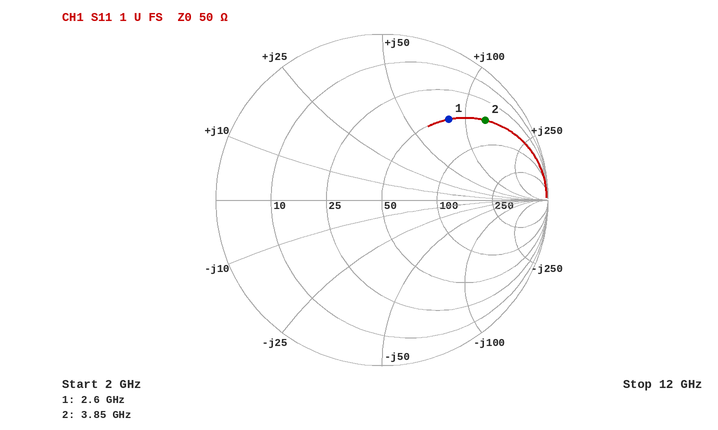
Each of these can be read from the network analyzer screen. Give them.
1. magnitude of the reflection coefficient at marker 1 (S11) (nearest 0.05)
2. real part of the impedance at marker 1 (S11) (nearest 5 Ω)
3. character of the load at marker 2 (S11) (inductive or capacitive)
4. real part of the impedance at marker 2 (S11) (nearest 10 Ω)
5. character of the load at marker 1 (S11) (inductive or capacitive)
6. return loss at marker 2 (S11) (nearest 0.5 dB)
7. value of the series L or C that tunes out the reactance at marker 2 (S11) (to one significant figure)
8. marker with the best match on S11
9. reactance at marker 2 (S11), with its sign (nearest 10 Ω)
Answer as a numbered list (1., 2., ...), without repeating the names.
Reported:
1. 0.65
2. 50 Ω
3. inductive
4. 50 Ω
5. inductive
6. 2.0 dB
7. 300 fF
8. marker 1
9. +130 Ω
